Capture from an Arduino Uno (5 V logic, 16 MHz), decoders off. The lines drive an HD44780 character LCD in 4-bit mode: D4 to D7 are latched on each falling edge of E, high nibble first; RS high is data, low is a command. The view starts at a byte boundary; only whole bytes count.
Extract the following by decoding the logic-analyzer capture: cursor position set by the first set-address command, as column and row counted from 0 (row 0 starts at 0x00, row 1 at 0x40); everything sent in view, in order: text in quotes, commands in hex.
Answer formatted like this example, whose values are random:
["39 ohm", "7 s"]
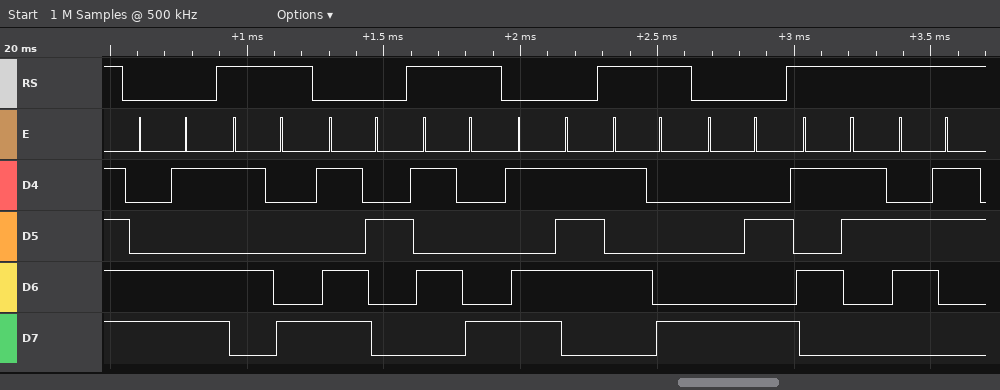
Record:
["column 13, row 1", "0xCD \"X\" 0xD2 \"X\" 0xD7 \"X\" 0x8A \"Sc\""]
